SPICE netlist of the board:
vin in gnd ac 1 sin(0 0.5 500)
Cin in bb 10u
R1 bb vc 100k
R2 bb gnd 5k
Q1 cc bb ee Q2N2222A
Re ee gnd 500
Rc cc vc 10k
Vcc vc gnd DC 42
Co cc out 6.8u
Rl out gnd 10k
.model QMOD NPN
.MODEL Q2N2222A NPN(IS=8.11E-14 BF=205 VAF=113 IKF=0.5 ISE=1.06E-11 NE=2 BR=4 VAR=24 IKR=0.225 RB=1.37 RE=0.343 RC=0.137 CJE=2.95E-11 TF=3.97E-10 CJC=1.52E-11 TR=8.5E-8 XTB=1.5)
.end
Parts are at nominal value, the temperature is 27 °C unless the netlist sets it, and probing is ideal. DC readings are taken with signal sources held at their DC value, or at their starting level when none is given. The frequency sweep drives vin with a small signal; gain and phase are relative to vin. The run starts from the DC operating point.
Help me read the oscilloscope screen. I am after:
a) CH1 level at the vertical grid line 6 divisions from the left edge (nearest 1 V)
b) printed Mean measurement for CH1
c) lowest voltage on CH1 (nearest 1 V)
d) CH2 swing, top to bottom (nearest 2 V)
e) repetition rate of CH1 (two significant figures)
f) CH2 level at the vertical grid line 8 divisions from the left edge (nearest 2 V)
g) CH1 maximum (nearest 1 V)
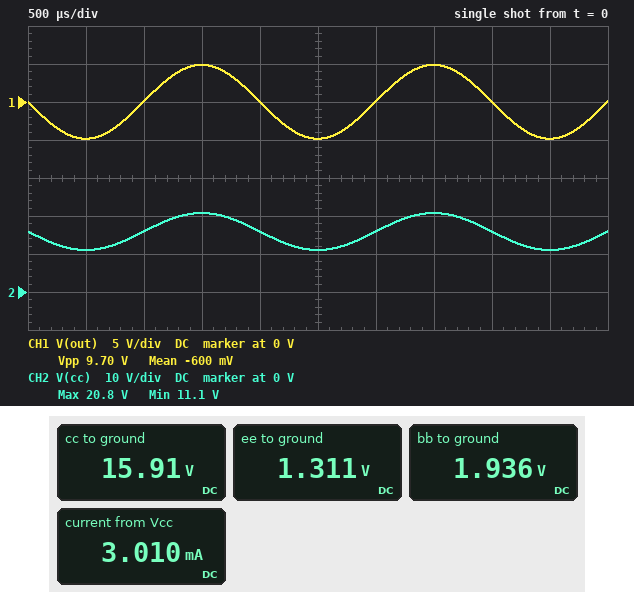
0 V
-600 mV
-5 V
10 V
500 Hz
16 V
5 V
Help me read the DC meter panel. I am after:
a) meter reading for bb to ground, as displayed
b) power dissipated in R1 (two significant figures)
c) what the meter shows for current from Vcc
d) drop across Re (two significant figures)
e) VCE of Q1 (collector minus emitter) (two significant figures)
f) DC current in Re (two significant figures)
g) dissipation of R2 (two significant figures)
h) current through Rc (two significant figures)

1.936 V
16 mW
3.010 mA
1.3 V
15 V
2.6 mA
750 µW
2.6 mA
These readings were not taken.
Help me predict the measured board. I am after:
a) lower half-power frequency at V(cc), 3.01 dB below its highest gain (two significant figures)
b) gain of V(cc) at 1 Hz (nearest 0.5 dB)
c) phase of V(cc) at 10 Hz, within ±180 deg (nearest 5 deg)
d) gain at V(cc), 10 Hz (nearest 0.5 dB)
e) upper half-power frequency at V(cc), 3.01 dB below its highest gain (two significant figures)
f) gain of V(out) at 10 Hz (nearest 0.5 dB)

2.4 Hz
13.0 dB
-165 deg
19.5 dB
5.7 MHz
19.0 dB
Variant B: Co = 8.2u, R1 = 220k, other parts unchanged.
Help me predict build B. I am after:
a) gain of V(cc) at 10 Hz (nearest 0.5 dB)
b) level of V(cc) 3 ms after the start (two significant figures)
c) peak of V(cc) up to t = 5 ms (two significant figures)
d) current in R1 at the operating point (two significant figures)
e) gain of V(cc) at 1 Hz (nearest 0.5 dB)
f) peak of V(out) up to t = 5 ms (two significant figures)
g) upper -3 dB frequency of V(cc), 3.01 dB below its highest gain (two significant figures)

19.0 dB
35 V
39 V
190 µA
12.0 dB
3.3 V
7.6 MHz
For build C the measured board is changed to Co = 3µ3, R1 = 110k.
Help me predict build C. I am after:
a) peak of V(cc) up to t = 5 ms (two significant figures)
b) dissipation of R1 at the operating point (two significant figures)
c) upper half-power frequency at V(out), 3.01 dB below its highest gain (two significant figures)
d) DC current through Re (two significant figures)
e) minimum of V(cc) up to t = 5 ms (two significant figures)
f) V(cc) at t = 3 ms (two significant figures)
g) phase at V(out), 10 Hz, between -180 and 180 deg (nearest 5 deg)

24 V
15 mW
6.1 MHz
2.3 mA
14 V
19 V
-145 deg
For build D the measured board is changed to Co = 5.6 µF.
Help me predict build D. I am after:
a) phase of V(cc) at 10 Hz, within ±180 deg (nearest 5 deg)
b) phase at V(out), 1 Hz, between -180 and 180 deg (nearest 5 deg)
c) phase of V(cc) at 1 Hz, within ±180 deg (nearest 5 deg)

-170 deg
-50 deg
-120 deg
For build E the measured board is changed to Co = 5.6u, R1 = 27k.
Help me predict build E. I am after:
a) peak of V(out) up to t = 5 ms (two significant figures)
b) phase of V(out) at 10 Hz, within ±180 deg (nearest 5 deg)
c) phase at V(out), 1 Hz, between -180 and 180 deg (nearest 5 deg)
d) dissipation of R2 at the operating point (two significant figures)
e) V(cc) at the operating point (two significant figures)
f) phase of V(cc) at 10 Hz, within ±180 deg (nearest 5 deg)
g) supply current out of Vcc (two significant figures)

1.0 V
90 deg
160 deg
1.9 mW
2.4 V
75 deg
5.4 mA
